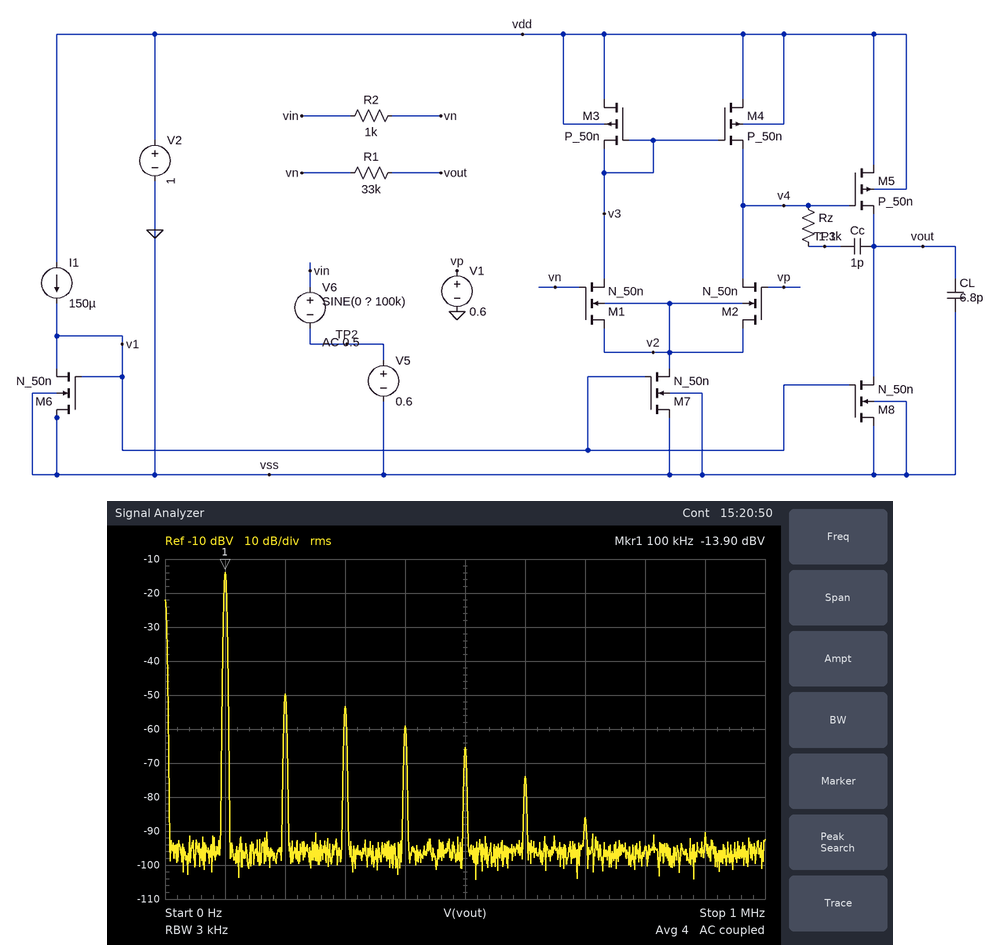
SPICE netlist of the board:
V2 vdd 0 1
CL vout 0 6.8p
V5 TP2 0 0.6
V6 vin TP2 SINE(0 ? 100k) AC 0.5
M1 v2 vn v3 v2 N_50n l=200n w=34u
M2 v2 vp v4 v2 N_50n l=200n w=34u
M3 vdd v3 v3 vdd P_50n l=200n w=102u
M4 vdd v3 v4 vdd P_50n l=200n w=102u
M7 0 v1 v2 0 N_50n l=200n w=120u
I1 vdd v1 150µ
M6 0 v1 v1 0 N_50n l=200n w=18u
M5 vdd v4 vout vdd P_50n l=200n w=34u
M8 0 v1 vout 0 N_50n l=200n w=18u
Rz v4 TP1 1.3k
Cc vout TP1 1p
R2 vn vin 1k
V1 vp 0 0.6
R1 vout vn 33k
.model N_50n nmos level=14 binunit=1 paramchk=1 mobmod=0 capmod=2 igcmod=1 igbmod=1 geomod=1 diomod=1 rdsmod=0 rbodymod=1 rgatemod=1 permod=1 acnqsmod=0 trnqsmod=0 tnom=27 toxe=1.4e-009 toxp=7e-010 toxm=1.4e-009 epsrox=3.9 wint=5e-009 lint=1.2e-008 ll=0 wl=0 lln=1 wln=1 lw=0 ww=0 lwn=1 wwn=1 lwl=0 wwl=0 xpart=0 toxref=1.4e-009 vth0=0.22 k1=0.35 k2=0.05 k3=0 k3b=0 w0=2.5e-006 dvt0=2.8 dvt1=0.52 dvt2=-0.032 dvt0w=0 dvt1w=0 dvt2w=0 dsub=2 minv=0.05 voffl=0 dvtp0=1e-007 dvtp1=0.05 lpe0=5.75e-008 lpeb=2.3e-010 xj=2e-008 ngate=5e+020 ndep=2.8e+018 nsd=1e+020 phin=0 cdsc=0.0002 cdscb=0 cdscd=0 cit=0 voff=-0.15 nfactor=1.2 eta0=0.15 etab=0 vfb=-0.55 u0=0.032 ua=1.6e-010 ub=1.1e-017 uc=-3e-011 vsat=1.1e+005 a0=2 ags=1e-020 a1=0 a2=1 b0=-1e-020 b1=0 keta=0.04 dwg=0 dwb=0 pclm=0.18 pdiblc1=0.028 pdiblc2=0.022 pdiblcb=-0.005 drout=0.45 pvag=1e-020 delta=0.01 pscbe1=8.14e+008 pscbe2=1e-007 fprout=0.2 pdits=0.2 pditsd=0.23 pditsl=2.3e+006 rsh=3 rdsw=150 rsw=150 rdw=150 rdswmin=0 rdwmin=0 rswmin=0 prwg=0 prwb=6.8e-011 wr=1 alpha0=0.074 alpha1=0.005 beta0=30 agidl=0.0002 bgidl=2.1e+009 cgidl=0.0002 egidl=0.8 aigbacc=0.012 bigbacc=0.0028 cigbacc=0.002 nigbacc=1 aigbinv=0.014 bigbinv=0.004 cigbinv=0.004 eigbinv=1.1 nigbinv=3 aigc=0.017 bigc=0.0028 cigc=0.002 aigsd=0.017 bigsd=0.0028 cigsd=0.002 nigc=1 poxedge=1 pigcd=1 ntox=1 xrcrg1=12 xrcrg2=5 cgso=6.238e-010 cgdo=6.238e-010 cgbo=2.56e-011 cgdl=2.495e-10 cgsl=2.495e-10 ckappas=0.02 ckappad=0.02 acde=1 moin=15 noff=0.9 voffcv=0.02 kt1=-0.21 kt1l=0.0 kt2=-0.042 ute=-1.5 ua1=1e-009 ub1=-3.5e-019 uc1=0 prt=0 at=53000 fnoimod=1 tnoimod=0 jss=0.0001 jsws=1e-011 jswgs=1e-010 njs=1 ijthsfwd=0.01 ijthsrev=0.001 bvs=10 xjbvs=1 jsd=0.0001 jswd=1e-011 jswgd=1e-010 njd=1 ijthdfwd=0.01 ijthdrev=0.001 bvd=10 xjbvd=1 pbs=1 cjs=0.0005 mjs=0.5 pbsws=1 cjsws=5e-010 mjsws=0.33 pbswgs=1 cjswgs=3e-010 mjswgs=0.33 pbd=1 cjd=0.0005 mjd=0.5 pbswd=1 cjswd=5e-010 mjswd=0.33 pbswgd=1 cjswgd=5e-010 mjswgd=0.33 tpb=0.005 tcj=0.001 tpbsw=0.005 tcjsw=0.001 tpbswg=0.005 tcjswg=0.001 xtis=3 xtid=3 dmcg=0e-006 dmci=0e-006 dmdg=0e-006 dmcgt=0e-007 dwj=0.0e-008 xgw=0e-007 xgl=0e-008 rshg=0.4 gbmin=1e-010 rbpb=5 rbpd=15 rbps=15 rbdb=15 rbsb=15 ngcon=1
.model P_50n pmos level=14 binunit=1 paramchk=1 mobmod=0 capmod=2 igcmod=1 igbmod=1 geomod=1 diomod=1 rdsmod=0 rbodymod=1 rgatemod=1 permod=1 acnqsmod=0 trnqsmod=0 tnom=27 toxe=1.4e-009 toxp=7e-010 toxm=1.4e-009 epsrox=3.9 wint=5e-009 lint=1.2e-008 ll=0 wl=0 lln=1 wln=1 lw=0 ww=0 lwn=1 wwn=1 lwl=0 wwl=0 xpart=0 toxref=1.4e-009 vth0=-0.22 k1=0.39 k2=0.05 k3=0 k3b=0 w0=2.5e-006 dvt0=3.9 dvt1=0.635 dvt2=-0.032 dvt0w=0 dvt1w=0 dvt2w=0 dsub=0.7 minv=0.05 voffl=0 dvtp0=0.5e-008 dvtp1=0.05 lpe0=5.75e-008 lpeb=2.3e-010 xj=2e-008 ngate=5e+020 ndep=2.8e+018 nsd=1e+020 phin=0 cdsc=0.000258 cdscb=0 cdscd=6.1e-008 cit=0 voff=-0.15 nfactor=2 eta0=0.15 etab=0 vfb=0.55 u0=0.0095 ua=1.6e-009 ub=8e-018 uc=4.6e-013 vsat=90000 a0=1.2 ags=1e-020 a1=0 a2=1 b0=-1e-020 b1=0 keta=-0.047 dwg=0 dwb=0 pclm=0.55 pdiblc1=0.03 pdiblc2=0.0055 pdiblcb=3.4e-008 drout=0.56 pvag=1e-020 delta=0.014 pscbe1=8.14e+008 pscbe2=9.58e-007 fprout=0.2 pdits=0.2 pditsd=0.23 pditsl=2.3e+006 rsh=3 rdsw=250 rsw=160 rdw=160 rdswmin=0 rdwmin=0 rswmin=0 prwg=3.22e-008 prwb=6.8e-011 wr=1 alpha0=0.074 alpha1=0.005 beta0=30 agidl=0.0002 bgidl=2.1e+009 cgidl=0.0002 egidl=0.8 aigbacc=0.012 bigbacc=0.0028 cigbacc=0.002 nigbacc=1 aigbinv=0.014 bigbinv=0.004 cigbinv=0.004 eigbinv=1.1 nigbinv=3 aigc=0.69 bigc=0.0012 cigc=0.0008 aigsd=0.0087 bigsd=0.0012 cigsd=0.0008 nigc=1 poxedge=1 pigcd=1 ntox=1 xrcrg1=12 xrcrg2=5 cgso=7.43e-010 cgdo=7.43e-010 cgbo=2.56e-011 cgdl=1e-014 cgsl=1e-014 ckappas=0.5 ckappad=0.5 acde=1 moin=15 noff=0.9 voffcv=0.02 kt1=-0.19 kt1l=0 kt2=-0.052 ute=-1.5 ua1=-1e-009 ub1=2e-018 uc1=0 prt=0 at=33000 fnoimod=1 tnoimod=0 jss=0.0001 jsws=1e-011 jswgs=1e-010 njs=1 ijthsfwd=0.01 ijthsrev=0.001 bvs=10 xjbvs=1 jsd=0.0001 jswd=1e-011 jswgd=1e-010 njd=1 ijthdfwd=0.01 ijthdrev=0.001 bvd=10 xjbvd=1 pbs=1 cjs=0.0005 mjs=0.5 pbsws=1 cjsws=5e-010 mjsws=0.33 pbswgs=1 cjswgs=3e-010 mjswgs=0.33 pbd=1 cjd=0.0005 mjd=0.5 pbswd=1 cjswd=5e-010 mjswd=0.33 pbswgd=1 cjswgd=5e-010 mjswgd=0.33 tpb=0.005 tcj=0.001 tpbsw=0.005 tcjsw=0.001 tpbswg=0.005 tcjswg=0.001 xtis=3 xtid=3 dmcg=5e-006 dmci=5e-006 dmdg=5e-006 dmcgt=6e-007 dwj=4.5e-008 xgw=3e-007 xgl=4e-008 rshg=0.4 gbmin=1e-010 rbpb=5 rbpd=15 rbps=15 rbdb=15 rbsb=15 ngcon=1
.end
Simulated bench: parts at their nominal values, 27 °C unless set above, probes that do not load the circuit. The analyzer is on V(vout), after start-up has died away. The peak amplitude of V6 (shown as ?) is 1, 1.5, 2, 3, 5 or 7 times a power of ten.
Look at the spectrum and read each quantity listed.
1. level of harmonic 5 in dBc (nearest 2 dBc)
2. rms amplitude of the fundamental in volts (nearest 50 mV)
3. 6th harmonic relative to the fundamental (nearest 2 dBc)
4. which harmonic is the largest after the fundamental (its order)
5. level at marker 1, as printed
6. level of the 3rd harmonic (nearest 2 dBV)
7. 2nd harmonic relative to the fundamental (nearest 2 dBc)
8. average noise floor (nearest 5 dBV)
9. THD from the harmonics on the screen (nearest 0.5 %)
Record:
-52 dBc
200 mV
-60 dBc
2
-13.90 dBV
-54 dBV
-36 dBc
-95 dBV
2.0 %
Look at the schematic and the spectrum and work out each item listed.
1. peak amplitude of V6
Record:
10 mV
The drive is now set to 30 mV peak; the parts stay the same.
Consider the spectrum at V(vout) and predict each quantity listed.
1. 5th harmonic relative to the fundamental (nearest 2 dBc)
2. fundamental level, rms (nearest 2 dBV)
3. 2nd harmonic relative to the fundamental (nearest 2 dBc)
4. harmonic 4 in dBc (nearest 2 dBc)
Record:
-32 dBc
-8 dBV
-20 dBc
-28 dBc
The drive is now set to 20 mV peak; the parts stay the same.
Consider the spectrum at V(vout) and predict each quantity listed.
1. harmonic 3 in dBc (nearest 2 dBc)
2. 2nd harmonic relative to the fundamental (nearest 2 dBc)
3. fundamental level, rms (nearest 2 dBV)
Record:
-22 dBc
-20 dBc
-10 dBV
